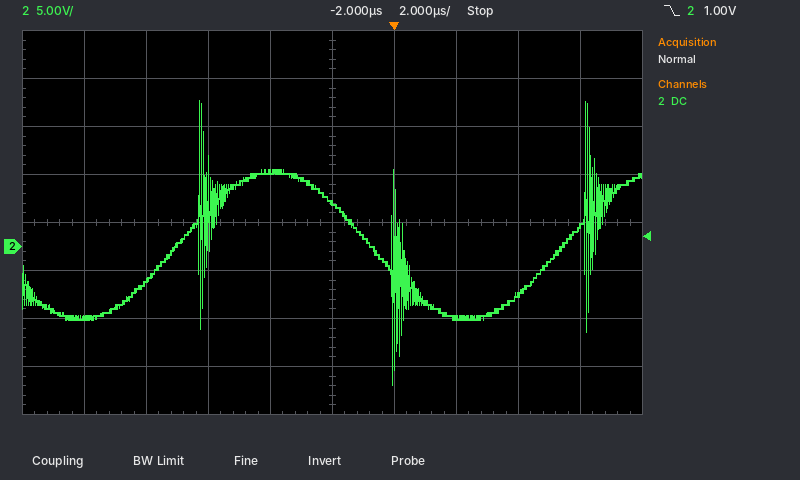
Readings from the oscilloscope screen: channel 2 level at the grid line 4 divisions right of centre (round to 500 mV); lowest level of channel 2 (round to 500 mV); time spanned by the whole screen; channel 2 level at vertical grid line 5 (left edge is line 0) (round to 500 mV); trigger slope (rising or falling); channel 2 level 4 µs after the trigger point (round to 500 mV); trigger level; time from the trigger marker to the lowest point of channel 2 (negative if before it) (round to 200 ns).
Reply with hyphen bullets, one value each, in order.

- 2.0 V
- -14.5 V
- 20 µs
- 4.5 V
- falling
- -5.0 V
- 1.00 V
- 0.0 µs
